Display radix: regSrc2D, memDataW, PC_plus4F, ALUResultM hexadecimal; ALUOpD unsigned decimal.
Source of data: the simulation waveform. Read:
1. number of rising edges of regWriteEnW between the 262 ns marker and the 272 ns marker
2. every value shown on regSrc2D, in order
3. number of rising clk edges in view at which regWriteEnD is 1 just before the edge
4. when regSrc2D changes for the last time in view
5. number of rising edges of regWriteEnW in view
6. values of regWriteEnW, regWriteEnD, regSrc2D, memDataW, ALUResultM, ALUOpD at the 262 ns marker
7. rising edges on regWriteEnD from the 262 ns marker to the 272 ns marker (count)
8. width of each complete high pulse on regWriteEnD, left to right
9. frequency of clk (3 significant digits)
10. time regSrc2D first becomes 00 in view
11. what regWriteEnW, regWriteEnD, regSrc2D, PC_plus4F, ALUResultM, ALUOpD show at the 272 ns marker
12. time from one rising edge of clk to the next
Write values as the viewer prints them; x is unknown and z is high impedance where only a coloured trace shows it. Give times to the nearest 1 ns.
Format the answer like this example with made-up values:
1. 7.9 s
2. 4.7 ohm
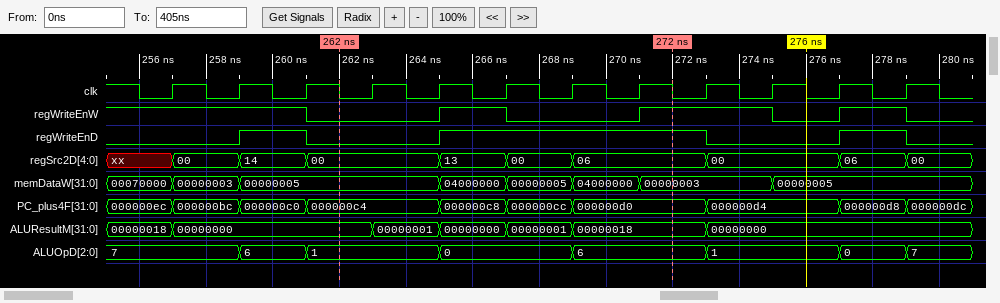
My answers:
1. 2
2. xx, 00, 14, 00, 13, 00, 06, 00, 06, 00
3. 6
4. 279 ns
5. 3
6. regWriteEnW=0, regWriteEnD=0, regSrc2D=00, memDataW=00000005, ALUResultM=00000000, ALUOpD=1
7. 1
8. 2 ns, 8 ns, 2 ns
9. 500 MHz
10. 257 ns
11. regWriteEnW=1, regWriteEnD=1, regSrc2D=06, PC_plus4F=000000d0, ALUResultM=00000018, ALUOpD=6
12. 2 ns
